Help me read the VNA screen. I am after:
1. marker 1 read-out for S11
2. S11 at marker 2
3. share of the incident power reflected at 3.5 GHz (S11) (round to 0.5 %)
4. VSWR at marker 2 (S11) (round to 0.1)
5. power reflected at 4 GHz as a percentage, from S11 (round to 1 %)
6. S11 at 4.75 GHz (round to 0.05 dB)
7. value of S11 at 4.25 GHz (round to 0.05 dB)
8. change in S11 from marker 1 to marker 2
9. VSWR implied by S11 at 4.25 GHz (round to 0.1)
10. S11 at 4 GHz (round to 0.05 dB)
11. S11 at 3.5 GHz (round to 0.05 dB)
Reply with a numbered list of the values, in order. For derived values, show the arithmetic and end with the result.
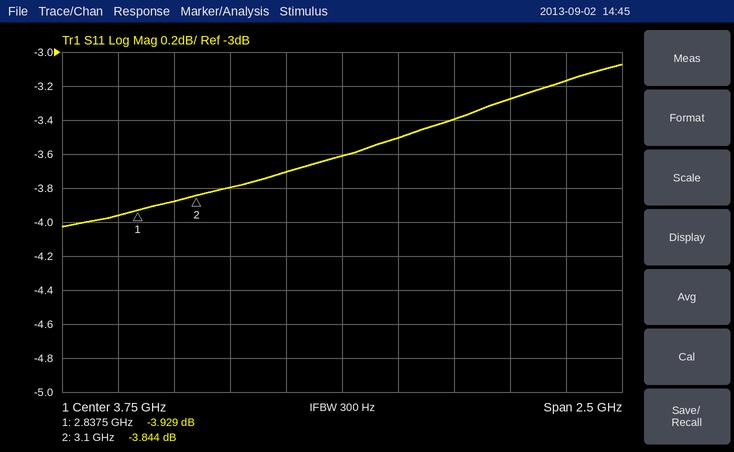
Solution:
1. -3.929 dB
2. -3.844 dB
3. 10^(-3.7/10) ≈ 42.7 %, so 42.5 % to the nearest 0.5 %
4. (1 + 0.6424)/(1 − 0.6424) ≈ 4.6
5. 10^(-3.5/10) ≈ 45 %
6. -3.15 dB
7. -3.40 dB
8. -3.844 − (-3.929) = 0.085 dB
9. |Γ| = 10^(-3.4/20) = 0.6761; VSWR = (1 + 0.6761)/(1 − 0.6761) ≈ 5.2
10. -3.50 dB
11. -3.70 dB
